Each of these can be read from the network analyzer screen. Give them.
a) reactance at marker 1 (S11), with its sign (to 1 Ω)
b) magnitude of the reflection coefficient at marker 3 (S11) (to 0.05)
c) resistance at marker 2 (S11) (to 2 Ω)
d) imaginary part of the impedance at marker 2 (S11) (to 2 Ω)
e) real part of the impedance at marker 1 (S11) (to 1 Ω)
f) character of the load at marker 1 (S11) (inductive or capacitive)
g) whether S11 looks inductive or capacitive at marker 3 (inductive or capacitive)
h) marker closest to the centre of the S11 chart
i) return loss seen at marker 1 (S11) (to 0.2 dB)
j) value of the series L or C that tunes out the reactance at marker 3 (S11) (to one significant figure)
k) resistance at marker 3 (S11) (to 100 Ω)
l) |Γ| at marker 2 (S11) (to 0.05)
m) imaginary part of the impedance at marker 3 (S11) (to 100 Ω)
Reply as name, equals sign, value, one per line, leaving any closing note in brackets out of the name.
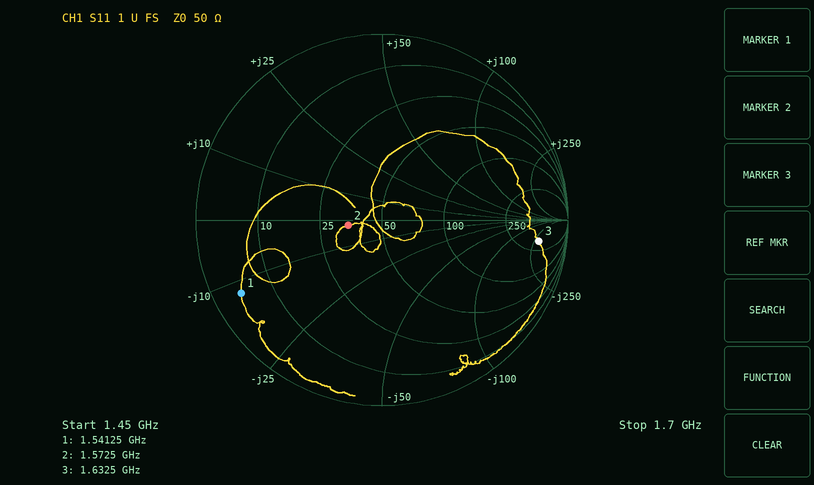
reactance at marker 1 (S11), with its sign = -12 Ω
magnitude of the reflection coefficient at marker 3 (S11) = 0.85
resistance at marker 2 (S11) = 34 Ω
imaginary part of the impedance at marker 2 (S11) = -2 Ω
real part of the impedance at marker 1 (S11) = 4 Ω
character of the load at marker 1 (S11) = capacitive
whether S11 looks inductive or capacitive at marker 3 = capacitive
marker closest to the centre of the S11 chart = marker 2
return loss seen at marker 1 (S11) = 1.4 dB
value of the series L or C that tunes out the reactance at marker 3 (S11) = 30 nH
resistance at marker 3 (S11) = 400 Ω
|Γ| at marker 2 (S11) = 0.20
imaginary part of the impedance at marker 3 (S11) = -300 Ω
